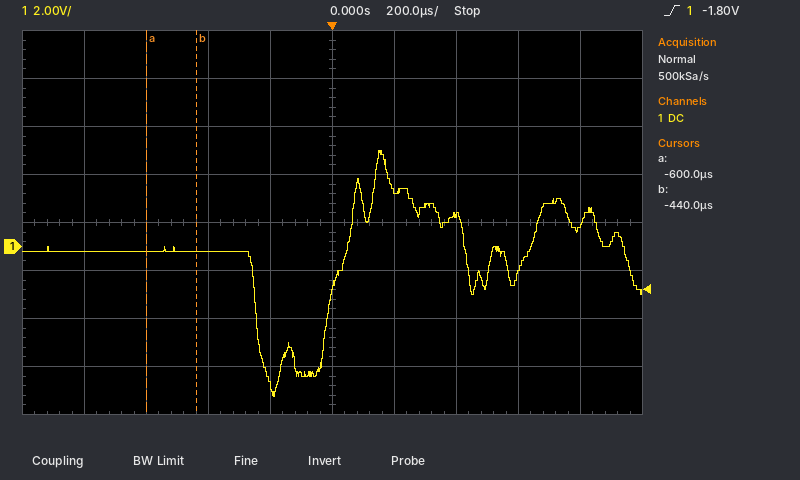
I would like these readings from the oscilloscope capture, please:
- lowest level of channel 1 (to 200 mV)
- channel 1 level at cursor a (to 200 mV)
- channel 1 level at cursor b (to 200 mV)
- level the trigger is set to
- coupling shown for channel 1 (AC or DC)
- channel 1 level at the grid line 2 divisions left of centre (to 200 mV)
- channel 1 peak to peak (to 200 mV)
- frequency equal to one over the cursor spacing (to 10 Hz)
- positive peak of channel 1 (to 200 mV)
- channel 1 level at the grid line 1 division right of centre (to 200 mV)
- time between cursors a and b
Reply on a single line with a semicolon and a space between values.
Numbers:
-6.2 V; -200 mV; -200 mV; -1.80 V; DC; -200 mV; 10.2 V; 6.25 kHz; 4.0 V; 2.4 V; 160 µs
